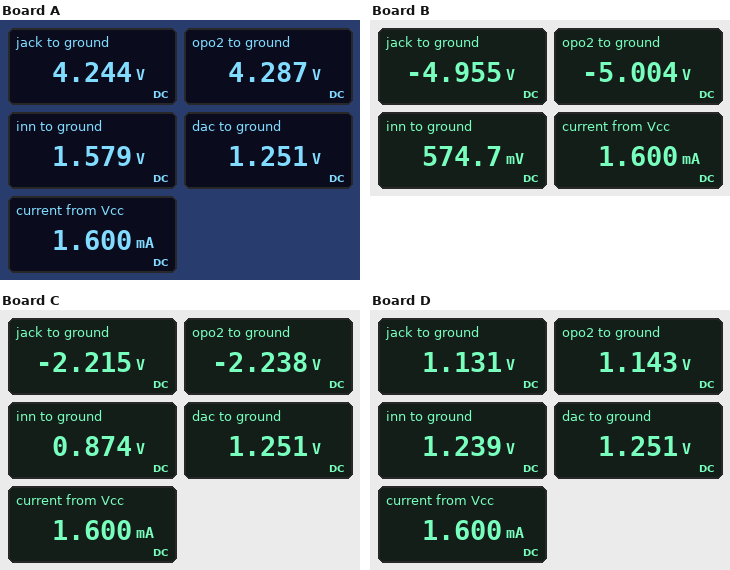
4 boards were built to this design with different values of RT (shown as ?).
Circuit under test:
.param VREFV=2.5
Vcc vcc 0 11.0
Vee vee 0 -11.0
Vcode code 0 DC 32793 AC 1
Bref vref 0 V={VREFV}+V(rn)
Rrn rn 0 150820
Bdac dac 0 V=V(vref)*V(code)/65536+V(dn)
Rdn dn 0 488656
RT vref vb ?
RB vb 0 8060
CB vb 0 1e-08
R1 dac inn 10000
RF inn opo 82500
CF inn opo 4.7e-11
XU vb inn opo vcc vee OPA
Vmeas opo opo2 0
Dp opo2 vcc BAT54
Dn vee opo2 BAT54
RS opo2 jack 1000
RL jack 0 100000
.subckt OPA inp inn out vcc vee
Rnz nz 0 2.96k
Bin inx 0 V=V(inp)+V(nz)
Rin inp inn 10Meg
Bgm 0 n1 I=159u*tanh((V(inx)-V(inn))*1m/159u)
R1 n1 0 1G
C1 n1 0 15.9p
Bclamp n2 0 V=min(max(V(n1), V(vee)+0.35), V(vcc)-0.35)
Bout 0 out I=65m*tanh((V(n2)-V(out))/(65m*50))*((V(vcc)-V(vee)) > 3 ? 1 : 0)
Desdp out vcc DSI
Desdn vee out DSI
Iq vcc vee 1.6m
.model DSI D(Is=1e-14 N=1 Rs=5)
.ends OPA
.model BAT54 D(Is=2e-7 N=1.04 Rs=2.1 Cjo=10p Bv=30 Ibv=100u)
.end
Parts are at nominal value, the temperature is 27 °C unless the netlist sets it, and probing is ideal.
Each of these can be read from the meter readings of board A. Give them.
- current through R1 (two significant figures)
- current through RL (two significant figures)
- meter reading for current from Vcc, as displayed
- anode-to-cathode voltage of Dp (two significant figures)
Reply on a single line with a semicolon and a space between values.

33 µA; 42 µA; 1.600 mA; -6.7 V
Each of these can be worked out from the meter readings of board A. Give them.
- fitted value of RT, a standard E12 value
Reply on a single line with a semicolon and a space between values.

4.7 kΩ
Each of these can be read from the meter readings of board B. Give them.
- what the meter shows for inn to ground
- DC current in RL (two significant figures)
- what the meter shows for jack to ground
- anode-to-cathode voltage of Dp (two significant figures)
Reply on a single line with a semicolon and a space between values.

574.7 mV; 50 µA; -4.955 V; -16 V
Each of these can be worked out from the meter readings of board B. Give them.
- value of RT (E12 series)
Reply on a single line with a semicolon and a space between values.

27 kΩ
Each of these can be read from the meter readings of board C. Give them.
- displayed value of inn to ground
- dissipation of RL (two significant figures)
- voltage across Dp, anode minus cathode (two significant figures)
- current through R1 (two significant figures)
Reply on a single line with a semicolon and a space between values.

0.874 V; 49 µW; -13 V; 38 µA
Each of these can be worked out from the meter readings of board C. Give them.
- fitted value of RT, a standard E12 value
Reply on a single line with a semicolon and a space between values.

15 kΩ
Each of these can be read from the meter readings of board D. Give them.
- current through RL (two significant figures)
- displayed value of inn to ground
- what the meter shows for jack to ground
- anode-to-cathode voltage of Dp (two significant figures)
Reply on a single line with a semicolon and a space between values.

11 µA; 1.239 V; 1.131 V; -9.9 V
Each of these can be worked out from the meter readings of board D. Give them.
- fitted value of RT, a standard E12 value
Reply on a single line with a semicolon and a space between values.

8.2 kΩ
